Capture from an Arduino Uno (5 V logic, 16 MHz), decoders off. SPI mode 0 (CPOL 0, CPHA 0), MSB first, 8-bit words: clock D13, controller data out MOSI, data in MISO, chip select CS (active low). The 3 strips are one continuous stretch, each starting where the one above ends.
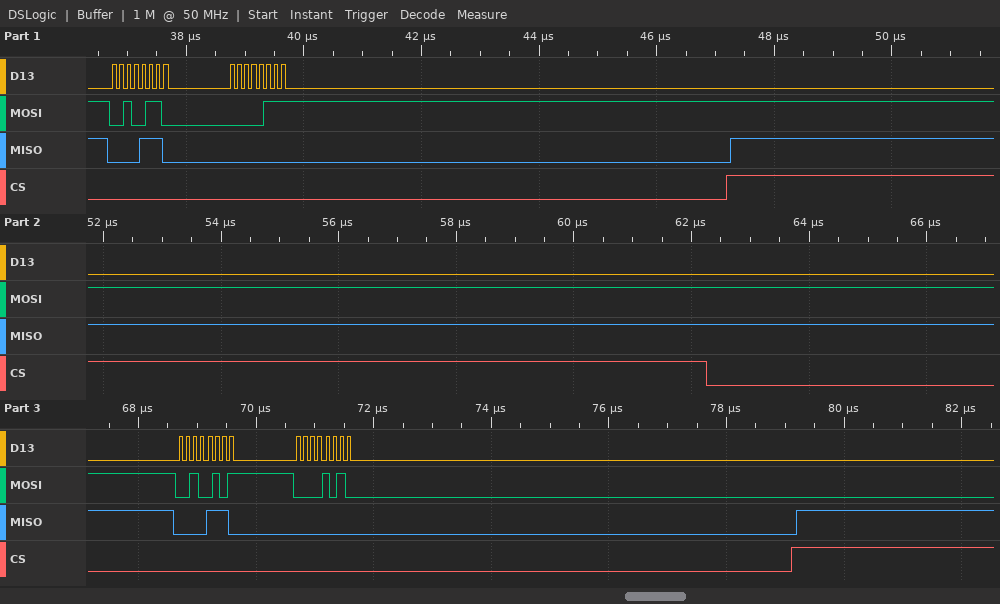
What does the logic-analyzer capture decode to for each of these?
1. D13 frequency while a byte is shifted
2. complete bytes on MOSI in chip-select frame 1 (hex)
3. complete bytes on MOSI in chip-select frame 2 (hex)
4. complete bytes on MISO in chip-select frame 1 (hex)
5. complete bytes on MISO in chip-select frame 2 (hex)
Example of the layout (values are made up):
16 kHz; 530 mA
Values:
8 MHz; 0x26 0x07; 0x25 0x0A; 0x0E 0x00; 0x0E 0x00
